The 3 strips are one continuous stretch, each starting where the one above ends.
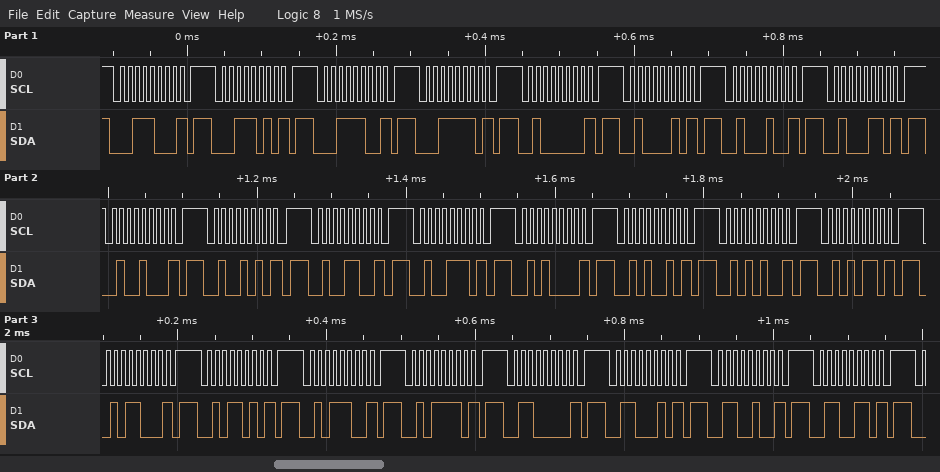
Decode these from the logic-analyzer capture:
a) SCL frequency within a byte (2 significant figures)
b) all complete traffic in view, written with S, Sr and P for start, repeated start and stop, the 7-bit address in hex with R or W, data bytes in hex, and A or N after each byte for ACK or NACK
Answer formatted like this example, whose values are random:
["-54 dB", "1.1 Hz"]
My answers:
["100 kHz", "S 1CW N P S 1DW N P S 1EW N P S 1FW N P S 20W N P S 21W N P S 22W N P S 23W N P S 24W N P S 25W N P S 26W N P S 27W N P S 28W N P S 29W N P S 2AW N P S 2BW N P S 2CW N P S 2DW N P S 2EW N P S 2FW N P S 30W N P S 31W N P S 32W N P S 33W N P"]
